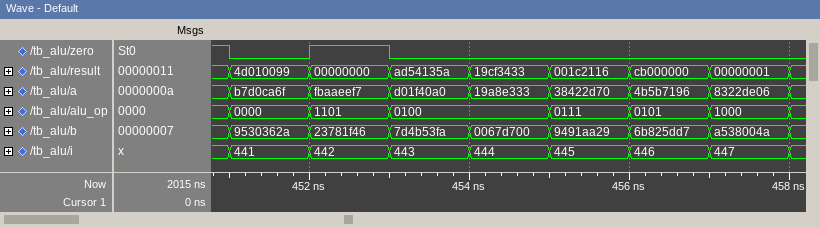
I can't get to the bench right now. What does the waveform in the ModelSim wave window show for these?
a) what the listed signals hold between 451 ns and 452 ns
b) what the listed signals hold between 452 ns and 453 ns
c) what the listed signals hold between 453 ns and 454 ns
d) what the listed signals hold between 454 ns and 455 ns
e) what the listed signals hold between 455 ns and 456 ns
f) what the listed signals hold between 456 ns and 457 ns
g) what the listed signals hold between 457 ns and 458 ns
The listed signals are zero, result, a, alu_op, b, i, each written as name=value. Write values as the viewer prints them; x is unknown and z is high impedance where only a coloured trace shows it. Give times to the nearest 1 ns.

zero=0, result=4d010099, a=b7d0ca6f, alu_op=0000, b=9530362a, i=441
zero=1, result=00000000, a=fbaaeef7, alu_op=1101, b=23781f46, i=442
zero=0, result=ad54135a, a=d01f40a0, alu_op=0100, b=7d4b53fa, i=443
zero=0, result=19cf3433, a=19a8e333, alu_op=0100, b=0067d700, i=444
zero=0, result=001c2116, a=38422d70, alu_op=0111, b=9491aa29, i=445
zero=0, result=cb000000, a=4b5b7196, alu_op=0101, b=6b825dd7, i=446
zero=0, result=00000001, a=8322de06, alu_op=1000, b=a538004a, i=447
